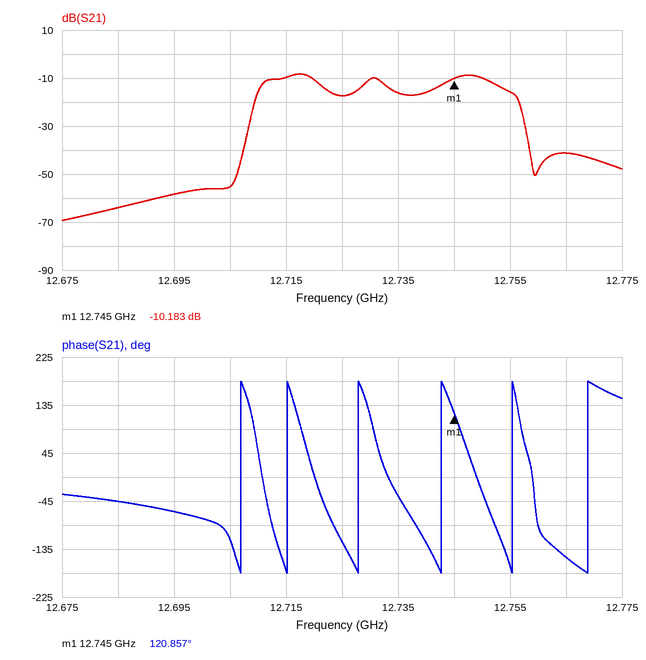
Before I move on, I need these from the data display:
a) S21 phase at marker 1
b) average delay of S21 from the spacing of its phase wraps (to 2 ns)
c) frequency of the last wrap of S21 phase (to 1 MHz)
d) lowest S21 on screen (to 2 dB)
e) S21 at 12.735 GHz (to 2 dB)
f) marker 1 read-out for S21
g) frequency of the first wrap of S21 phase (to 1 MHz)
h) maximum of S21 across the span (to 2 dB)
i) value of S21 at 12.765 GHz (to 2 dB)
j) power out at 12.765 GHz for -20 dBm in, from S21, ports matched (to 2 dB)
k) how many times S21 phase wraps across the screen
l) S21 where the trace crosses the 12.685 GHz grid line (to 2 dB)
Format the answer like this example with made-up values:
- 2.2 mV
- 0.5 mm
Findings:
- 120.857°
- 80 ns
- 12.769 GHz
- -70 dB
- -16 dB
- -10.183 dB
- 12.707 GHz
- -8 dB
- -42 dB
- -62 dBm
- 6
- -64 dB
